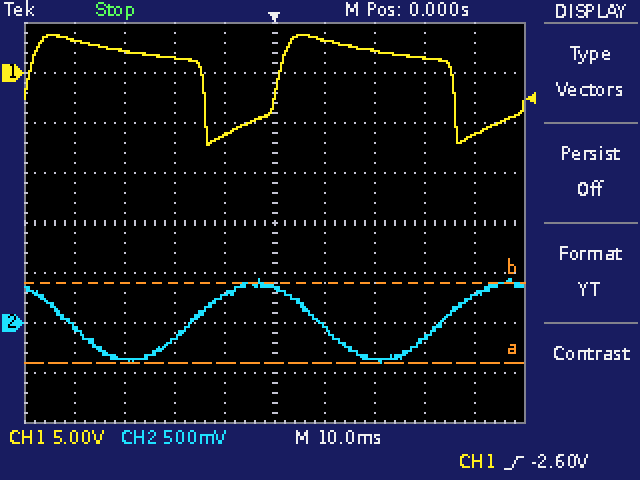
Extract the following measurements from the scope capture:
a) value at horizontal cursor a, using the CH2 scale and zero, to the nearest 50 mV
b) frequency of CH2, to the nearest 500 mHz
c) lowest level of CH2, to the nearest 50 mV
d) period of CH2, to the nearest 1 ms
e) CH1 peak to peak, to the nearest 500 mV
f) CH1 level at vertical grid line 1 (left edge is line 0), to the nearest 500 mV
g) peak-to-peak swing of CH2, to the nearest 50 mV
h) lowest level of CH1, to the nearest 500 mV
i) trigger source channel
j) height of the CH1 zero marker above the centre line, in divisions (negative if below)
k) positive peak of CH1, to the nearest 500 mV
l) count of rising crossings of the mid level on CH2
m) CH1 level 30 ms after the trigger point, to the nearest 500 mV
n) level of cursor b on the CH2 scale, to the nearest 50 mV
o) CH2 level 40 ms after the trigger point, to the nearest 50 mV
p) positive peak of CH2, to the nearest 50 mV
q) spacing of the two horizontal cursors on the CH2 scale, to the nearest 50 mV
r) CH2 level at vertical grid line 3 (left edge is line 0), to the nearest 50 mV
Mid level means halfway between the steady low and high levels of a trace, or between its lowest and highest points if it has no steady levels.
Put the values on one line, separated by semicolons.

-400 mV; 20.0 Hz; -400 mV; 50 ms; 11.0 V; 3.5 V; 850 mV; -7.0 V; CH1; +3.0 div; 4.0 V; 2; 1.5 V; 400 mV; 300 mV; 450 mV; 800 mV; -150 mV
